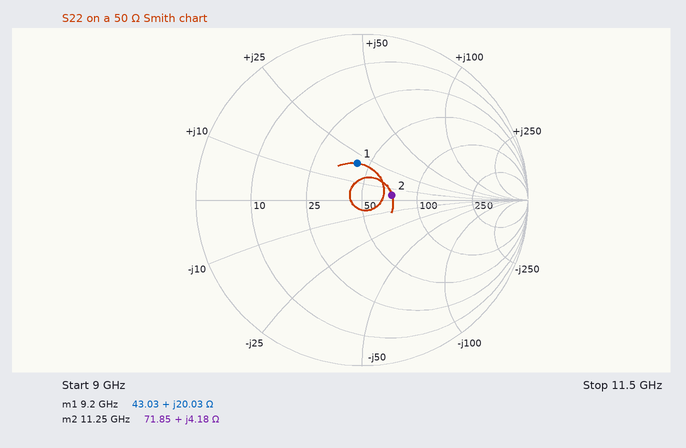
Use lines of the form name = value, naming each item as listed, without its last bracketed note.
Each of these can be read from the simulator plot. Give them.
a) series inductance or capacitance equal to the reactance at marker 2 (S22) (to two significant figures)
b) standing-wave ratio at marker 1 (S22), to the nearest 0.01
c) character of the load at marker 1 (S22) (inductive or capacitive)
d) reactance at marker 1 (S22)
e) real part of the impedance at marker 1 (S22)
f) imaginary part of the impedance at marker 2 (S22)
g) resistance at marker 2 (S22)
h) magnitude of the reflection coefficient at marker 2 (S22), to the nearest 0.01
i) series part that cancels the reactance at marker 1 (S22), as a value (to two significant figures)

series inductance or capacitance equal to the reactance at marker 2 (S22) = 59 pH
standing-wave ratio at marker 1 (S22), to the nearest 0.01 = 1.57
character of the load at marker 1 (S22) = inductive
reactance at marker 1 = +20.03 Ω
real part of the impedance at marker 1 = 43.03 Ω
imaginary part of the impedance at marker 2 = +4.18 Ω
resistance at marker 2 = 71.85 Ω
magnitude of the reflection coefficient at marker 2 (S22), to the nearest 0.01 = 0.18
series part that cancels the reactance at marker 1 (S22), as a value = 860 fF
